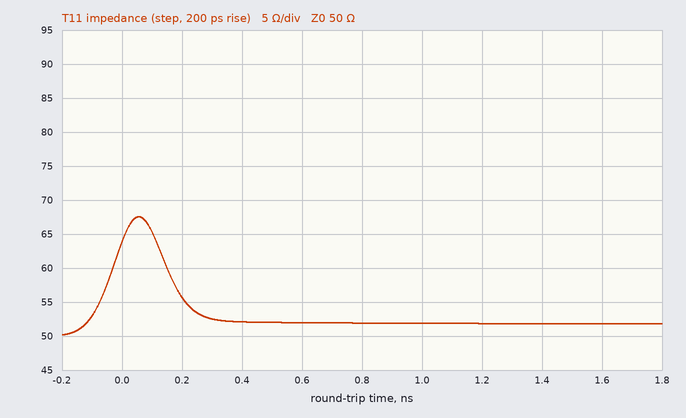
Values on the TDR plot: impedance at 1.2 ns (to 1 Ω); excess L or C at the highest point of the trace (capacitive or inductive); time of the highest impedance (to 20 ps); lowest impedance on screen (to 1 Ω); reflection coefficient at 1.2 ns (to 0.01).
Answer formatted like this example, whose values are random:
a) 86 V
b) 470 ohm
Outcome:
a) 52 Ω
b) inductive
c) 60 ps
d) 50 Ω
e) +0.02
